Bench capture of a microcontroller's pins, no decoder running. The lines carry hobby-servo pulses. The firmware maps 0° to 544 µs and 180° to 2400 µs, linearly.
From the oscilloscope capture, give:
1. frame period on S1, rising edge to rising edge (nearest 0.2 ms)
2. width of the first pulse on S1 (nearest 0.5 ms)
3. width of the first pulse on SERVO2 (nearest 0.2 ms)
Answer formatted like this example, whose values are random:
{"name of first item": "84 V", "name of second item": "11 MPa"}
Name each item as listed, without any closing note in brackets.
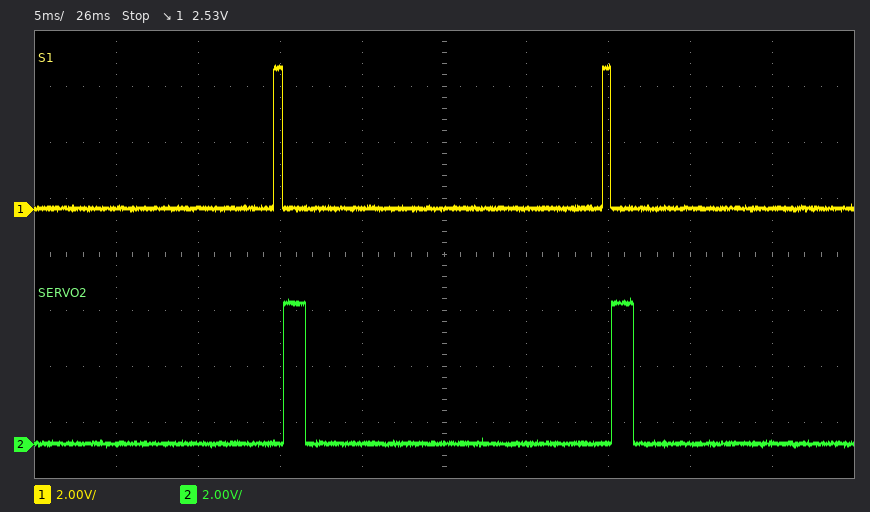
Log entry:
{"frame period on S1, rising edge to rising edge": "20.0 ms", "width of the first pulse on S1": "0.5 ms", "width of the first pulse on SERVO2": "1.4 ms"}
